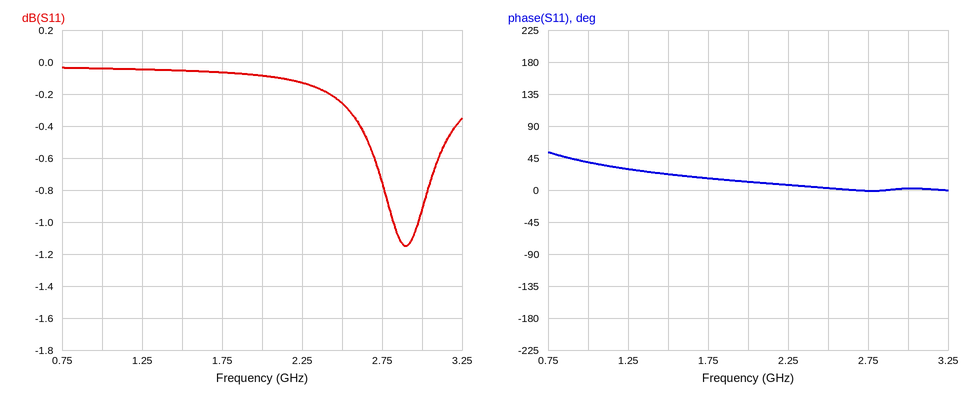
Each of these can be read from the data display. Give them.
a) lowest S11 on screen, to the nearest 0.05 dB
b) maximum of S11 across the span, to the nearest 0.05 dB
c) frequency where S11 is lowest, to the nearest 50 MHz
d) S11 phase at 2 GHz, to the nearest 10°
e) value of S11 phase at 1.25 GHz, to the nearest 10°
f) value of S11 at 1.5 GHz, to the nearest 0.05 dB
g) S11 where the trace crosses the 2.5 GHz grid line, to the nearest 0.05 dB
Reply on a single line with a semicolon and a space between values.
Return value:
-1.15 dB; -0.05 dB; 2.90 GHz; 10°; 30°; -0.05 dB; -0.25 dB
